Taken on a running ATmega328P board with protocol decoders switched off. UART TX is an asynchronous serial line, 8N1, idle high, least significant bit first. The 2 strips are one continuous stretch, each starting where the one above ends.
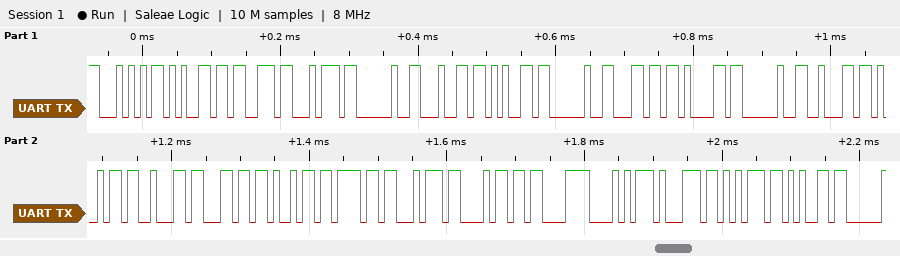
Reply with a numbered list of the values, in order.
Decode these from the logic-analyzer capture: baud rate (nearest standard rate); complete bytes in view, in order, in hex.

1. 115200 baud
2. 54 65 73 74 20 64 65 20 6C 61 20 62 69 62 6C 69 6F 74 68 C3 A8 71 75 65
